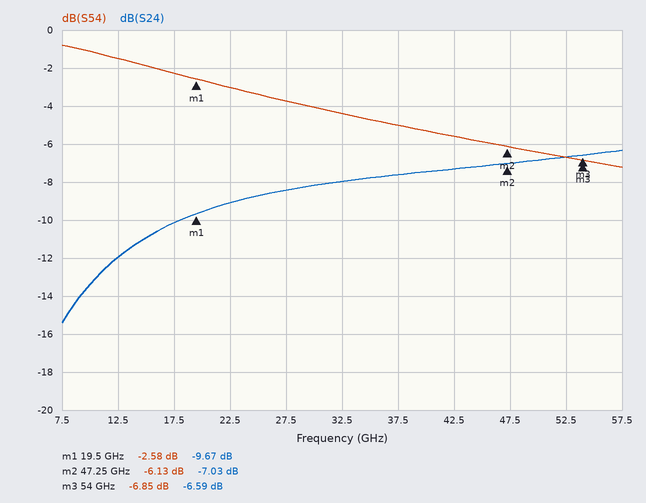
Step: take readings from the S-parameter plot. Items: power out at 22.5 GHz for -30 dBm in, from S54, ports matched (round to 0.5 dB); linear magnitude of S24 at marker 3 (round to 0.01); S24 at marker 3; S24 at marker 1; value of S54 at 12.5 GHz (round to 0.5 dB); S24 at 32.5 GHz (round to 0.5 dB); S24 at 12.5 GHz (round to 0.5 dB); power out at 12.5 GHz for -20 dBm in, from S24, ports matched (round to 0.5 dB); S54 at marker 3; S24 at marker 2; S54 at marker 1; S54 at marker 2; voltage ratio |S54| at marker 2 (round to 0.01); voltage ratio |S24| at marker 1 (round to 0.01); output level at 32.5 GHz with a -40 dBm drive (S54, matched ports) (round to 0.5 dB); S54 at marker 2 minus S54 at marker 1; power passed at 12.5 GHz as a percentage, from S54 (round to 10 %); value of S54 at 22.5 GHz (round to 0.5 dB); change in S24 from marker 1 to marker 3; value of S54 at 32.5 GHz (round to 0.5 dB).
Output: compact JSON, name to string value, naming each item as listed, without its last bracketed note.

{"power out at 22.5 GHz for -30 dBm in, from S54, ports matched": "-33.0 dBm", "linear magnitude of S24 at marker 3": "0.47", "S24 at marker 3": "-6.59 dB", "S24 at marker 1": "-9.67 dB", "value of S54 at 12.5 GHz": "-1.5 dB", "S24 at 32.5 GHz": "-8.0 dB", "S24 at 12.5 GHz": "-12.0 dB", "power out at 12.5 GHz for -20 dBm in, from S24, ports matched": "-32.0 dBm", "S54 at marker 3": "-6.85 dB", "S24 at marker 2": "-7.03 dB", "S54 at marker 1": "-2.58 dB", "S54 at marker 2": "-6.13 dB", "voltage ratio |S54| at marker 2": "0.49", "voltage ratio |S24| at marker 1": "0.33", "output level at 32.5 GHz with a -40 dBm drive (S54, matched ports)": "-44.5 dBm", "S54 at marker 2 minus S54 at marker 1": "-3.55 dB", "power passed at 12.5 GHz as a percentage, from S54": "70 %", "value of S54 at 22.5 GHz": "-3.0 dB", "change in S24 from marker 1 to marker 3": "3.08 dB", "value of S54 at 32.5 GHz": "-4.5 dB"}
